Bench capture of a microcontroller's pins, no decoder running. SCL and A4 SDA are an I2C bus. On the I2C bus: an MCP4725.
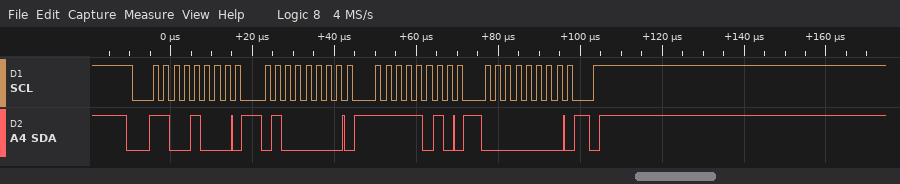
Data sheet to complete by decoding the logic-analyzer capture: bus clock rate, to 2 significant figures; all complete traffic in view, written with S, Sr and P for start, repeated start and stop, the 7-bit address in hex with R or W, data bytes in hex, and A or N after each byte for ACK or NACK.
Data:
400 kHz
S 64W A 40 A FA A 00 A P
